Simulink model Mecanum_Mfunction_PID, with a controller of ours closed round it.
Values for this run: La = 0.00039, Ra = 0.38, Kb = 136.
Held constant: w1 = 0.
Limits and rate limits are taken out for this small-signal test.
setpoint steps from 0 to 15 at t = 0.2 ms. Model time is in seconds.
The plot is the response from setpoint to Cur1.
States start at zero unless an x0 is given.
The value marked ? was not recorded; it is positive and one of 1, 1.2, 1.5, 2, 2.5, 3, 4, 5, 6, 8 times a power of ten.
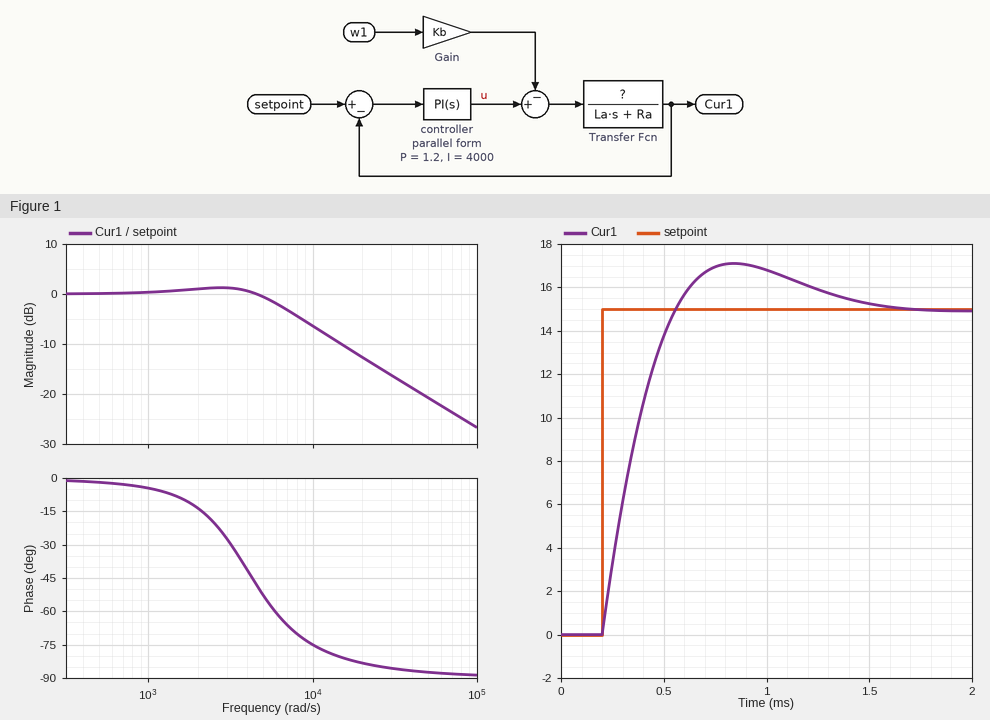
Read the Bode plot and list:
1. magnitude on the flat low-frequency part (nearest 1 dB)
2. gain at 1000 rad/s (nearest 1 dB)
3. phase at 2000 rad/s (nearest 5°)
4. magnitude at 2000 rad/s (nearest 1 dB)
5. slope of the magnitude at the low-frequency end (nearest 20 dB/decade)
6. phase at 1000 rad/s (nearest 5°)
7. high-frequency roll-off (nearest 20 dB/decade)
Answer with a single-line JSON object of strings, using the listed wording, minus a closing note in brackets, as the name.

{"magnitude on the flat low-frequency part": "0 dB", "gain at 1000 rad/s": "0 dB", "phase at 2000 rad/s": "-15°", "magnitude at 2000 rad/s": "1 dB", "slope of the magnitude at the low-frequency end": "0 dB/decade", "phase at 1000 rad/s": "-5°", "high-frequency roll-off": "-20 dB/decade"}
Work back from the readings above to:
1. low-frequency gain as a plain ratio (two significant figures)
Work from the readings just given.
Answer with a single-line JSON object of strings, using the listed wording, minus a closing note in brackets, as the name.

{"low-frequency gain as a plain ratio": "1.0"}
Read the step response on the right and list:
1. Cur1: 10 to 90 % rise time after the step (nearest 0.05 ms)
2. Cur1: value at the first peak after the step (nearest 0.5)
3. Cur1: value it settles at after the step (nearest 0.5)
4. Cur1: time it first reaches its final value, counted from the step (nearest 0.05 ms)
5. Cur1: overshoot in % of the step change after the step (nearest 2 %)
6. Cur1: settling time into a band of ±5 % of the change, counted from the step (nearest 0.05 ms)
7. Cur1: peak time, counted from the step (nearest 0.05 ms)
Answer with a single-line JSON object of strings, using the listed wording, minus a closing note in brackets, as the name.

{"Cur1: 10 to 90 % rise time after the step": "0.25 ms", "Cur1: value at the first peak after the step": "17.0", "Cur1: value it settles at after the step": "15.0", "Cur1: time it first reaches its final value, counted from the step": "0.35 ms", "Cur1: overshoot in % of the step change after the step": "14 %", "Cur1: settling time into a band of ±5 % of the change, counted from the step": "1.10 ms", "Cur1: peak time, counted from the step": "0.65 ms"}
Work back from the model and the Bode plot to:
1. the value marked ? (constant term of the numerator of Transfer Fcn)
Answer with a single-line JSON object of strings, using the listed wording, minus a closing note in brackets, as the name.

{"the value marked ?": "1.5"}
